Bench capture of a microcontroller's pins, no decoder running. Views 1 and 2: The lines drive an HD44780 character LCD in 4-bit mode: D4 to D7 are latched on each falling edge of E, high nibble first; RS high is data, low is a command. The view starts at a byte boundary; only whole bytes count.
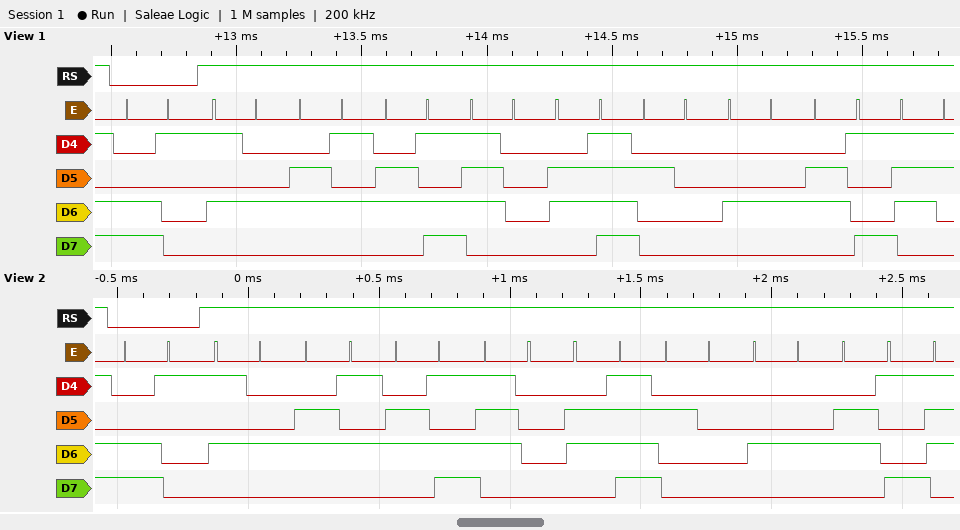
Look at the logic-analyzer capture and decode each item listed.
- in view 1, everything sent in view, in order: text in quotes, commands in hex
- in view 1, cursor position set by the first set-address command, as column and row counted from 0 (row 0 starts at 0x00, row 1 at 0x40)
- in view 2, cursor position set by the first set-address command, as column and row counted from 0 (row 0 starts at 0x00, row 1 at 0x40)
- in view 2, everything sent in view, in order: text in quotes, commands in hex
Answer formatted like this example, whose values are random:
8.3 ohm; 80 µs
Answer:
0xC1 "Tempo Dis"; column 1, row 1; column 1, row 1; 0xC1 "Tempo Di"
